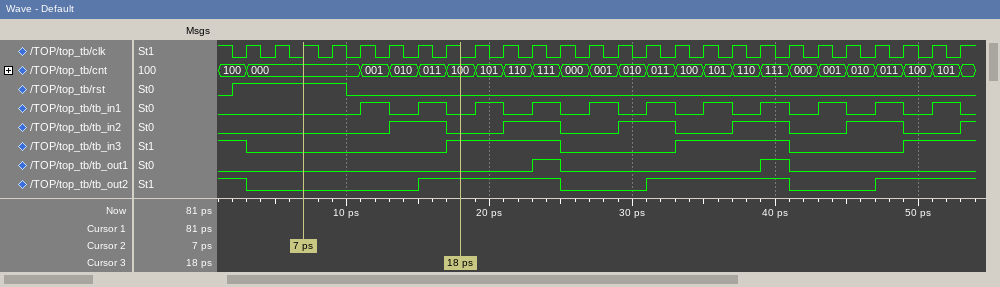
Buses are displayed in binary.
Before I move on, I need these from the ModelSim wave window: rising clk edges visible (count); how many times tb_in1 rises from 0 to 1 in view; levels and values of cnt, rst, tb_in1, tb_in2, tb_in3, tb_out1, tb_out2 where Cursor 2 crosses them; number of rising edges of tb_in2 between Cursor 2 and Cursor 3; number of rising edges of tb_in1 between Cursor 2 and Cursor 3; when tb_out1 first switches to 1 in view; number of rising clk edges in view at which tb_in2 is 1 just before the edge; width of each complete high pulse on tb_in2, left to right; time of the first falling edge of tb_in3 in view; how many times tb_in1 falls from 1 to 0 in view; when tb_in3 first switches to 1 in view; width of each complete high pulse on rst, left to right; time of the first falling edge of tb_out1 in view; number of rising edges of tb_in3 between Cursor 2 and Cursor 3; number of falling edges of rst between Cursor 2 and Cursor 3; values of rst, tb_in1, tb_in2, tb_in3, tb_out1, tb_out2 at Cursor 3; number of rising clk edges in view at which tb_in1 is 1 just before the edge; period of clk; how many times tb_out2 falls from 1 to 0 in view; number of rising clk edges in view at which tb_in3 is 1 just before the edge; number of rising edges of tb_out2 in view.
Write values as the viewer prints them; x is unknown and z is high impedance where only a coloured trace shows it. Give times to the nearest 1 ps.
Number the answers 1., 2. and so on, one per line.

1. 26
2. 11
3. cnt=000, rst=1, tb_in1=0, tb_in2=0, tb_in3=0, tb_out1=0, tb_out2=0
4. 1
5. 2
6. 23 ps
7. 10
8. 4 ps, 4 ps, 4 ps, 4 ps, 4 ps
9. 3 ps
10. 11
11. 17 ps
12. 8 ps
13. 25 ps
14. 1
15. 1
16. rst=0, tb_in1=0, tb_in2=0, tb_in3=1, tb_out1=0, tb_out2=1
17. 11
18. 2 ps
19. 3
20. 11
21. 3
